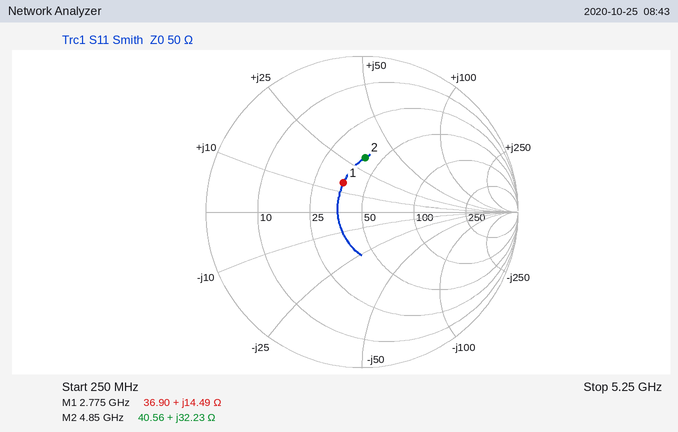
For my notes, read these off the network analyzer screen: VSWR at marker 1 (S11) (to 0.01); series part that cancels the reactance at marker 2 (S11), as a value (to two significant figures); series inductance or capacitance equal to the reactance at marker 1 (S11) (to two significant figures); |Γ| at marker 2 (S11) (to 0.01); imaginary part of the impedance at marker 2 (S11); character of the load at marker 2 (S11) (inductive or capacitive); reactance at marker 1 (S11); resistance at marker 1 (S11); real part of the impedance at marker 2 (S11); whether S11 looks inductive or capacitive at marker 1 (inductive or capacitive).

1.57
1.0 pF
830 pH
0.35
+32.23 Ω
inductive
+14.49 Ω
36.90 Ω
40.56 Ω
inductive
